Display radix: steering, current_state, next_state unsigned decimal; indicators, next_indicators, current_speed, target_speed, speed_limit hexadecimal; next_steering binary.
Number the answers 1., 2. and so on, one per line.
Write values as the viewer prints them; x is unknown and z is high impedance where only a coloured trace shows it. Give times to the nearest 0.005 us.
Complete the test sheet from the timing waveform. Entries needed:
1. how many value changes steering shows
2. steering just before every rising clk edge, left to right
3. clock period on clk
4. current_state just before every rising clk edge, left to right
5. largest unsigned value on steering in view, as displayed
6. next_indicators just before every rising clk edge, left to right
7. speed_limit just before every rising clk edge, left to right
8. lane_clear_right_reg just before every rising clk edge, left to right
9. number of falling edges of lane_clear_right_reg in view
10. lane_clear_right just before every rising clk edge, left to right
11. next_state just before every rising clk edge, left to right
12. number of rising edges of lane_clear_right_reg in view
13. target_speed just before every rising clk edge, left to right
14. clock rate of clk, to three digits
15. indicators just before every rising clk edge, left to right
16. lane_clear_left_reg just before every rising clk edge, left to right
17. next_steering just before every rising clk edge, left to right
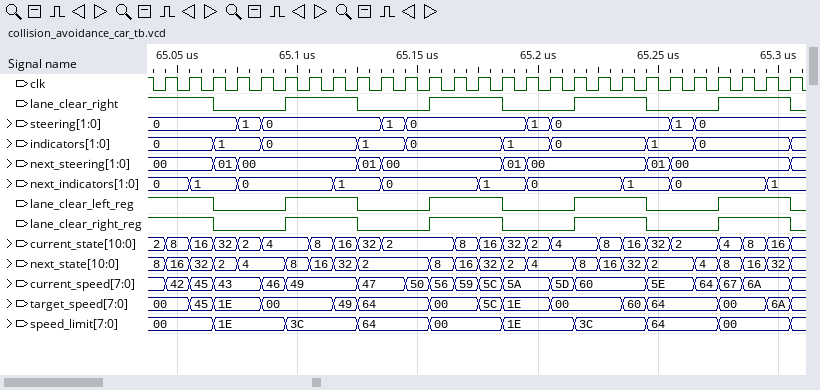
1. 8
2. 0, 0, 0, 0, 1, 0, 0, 0, 0, 0, 1, 0, 0, 0, 0, 0, 1, 0, 0, 0, 0, 0, 1, 0, 0, 0, 0
3. 0.01 us
4. 2, 8, 16, 32, 2, 4, 4, 8, 16, 32, 2, 2, 2, 8, 16, 32, 2, 4, 4, 8, 16, 32, 2, 2, 4, 8, 16
5. 1
6. 0, 0, 1, 1, 0, 0, 0, 0, 1, 1, 0, 0, 0, 0, 1, 1, 0, 0, 0, 0, 1, 1, 0, 0, 0, 0, 1
7. 00, 00, 00, 1E, 1E, 1E, 3C, 3C, 3C, 64, 64, 64, 00, 00, 00, 1E, 1E, 1E, 3C, 3C, 3C, 64, 64, 64, 00, 00, 00
8. 1 1 1 0 0 0 1 1 1 0 0 0 1 1 1 0 0 0 1 1 1 0 0 0 1 1 1
9. 5
10. 1 1 1 0 0 0 1 1 1 0 0 0 1 1 1 0 0 0 1 1 1 0 0 0 1 1 1
11. 8, 16, 32, 2, 4, 4, 8, 16, 32, 2, 2, 2, 8, 16, 32, 2, 4, 4, 8, 16, 32, 2, 2, 4, 8, 16, 32
12. 4
13. 00, 00, 45, 1E, 1E, 00, 00, 00, 49, 64, 64, 64, 00, 00, 5C, 1E, 1E, 00, 00, 00, 60, 64, 64, 64, 00, 00, 6A
14. 100 MHz
15. 0, 0, 0, 1, 1, 0, 0, 0, 0, 1, 1, 0, 0, 0, 0, 1, 1, 0, 0, 0, 0, 1, 1, 0, 0, 0, 0
16. 1 1 1 0 0 0 1 1 1 0 0 0 1 1 1 0 0 0 1 1 1 0 0 0 1 1 1
17. 00, 00, 00, 01, 00, 00, 00, 00, 00, 01, 00, 00, 00, 00, 00, 01, 00, 00, 00, 00, 00, 01, 00, 00, 00, 00, 00
